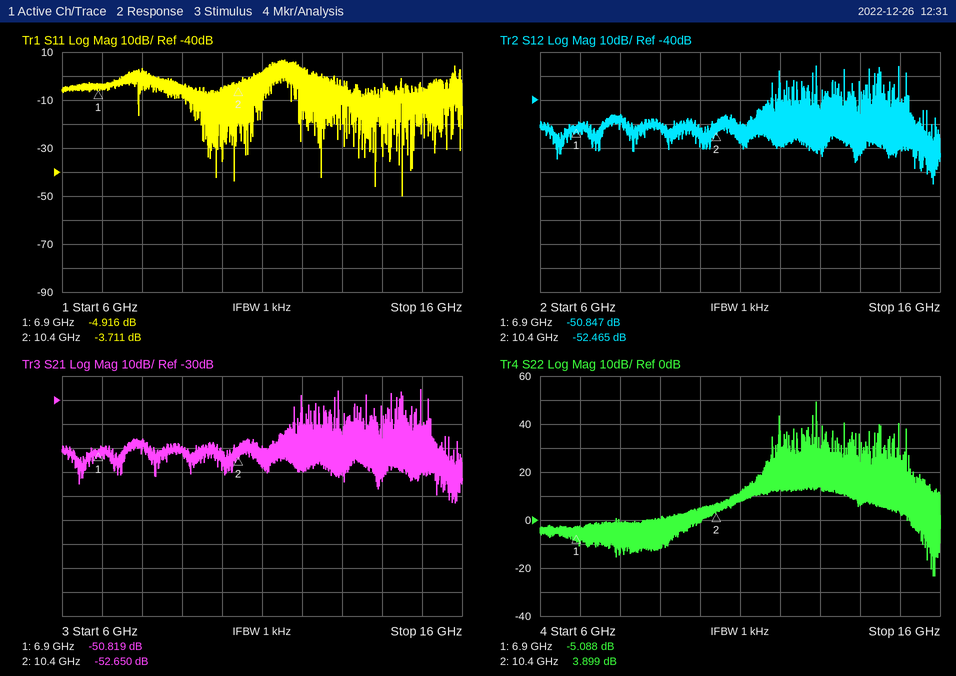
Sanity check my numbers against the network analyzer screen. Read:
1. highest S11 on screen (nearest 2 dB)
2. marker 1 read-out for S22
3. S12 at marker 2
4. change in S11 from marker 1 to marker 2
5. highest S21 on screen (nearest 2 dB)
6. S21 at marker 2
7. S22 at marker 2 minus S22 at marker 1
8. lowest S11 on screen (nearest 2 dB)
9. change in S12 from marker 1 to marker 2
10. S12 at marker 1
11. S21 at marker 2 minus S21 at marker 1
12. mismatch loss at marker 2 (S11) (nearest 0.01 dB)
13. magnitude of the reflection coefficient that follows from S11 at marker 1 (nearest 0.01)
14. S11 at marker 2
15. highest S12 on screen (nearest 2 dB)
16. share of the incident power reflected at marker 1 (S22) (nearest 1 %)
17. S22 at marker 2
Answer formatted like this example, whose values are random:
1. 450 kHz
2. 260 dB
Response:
1. 6 dB
2. -5.088 dB
3. -52.465 dB
4. 1.205 dB
5. -26 dB
6. -52.650 dB
7. 8.987 dB
8. -50 dB
9. -1.618 dB
10. -50.847 dB
11. -1.831 dB
12. 2.41 dB
13. 0.57
14. -3.711 dB
15. -26 dB
16. 31 %
17. 3.899 dB
